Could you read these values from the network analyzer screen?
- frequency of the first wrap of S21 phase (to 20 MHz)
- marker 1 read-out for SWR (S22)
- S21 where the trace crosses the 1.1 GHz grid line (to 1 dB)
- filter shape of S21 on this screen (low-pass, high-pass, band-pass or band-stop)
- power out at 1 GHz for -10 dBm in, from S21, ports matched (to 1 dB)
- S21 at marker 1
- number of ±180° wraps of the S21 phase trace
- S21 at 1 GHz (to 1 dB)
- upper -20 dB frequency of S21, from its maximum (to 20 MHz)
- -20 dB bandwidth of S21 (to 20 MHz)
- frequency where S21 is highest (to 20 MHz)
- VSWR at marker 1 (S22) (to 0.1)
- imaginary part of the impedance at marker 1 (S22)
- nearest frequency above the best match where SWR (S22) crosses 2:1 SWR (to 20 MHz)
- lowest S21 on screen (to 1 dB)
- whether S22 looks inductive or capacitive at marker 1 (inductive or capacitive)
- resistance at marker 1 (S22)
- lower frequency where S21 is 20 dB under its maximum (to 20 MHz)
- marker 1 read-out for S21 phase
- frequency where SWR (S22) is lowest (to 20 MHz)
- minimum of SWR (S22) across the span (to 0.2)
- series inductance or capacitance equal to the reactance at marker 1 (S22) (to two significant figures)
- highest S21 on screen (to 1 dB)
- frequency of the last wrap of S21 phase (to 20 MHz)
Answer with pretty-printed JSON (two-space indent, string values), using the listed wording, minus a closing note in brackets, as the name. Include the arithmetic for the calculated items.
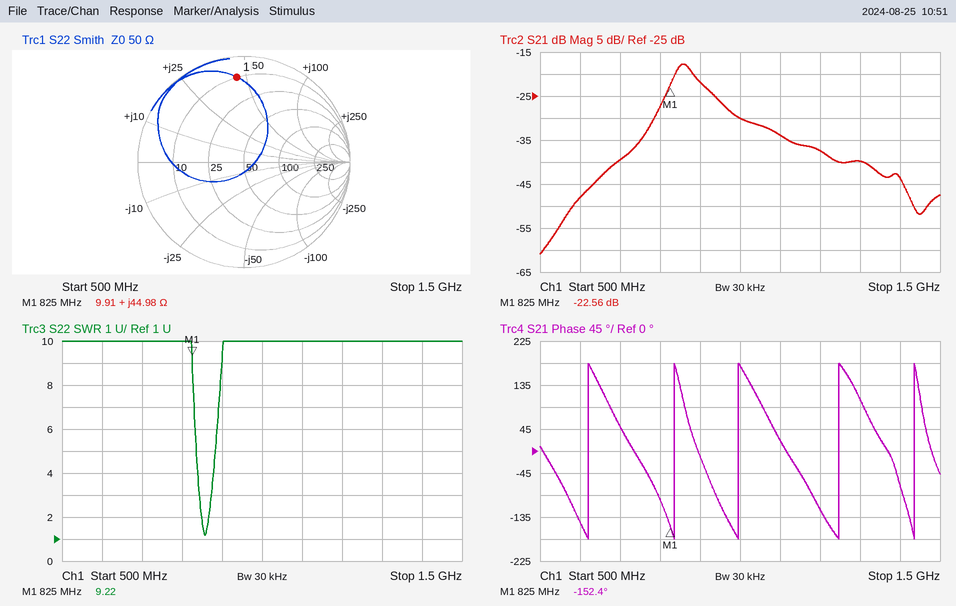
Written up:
{
  "frequency of the first wrap of S21 phase": "620 MHz",
  "marker 1 read-out for SWR": "9.22",
  "S21 where the trace crosses the 1.1 GHz grid line": "-34 dB",
  "filter shape of S21 on this screen": "band-pass",
  "power out at 1 GHz for -10 dBm in, from S21, ports matched": "-10 dBm + (-30 dB) = -40 dBm",
  "S21 at marker 1": "-22.56 dB",
  "number of ±180° wraps of the S21 phase trace": "5",
  "S21 at 1 GHz": "-30 dB",
  "upper -20 dB frequency of S21, from its maximum": "1.20 GHz",
  "-20 dB bandwidth of S21": "1.20 GHz − 720 MHz = 480 MHz",
  "frequency where S21 is highest": "860 MHz",
  "VSWR at marker 1 (S22)": "9.2",
  "imaginary part of the impedance at marker 1": "+44.98 Ω",
  "nearest frequency above the best match where SWR (S22) crosses 2:1 SWR": "860 MHz",
  "lowest S21 on screen": "-61 dB",
  "whether S22 looks inductive or capacitive at marker 1": "inductive",
  "resistance at marker 1": "9.91 Ω",
  "lower frequency where S21 is 20 dB under its maximum": "720 MHz",
  "marker 1 read-out for S21 phase": "-152.4°",
  "frequency where SWR (S22) is lowest": "860 MHz",
  "minimum of SWR (S22) across the span": "1.2",
  "series inductance or capacitance equal to the reactance at marker 1 (S22)": "L = 44.98 Ω/(2π × 825 MHz) ≈ 8.7 nH",
  "highest S21 on screen": "-18 dB",
  "frequency of the last wrap of S21 phase": "1.44 GHz"
}
